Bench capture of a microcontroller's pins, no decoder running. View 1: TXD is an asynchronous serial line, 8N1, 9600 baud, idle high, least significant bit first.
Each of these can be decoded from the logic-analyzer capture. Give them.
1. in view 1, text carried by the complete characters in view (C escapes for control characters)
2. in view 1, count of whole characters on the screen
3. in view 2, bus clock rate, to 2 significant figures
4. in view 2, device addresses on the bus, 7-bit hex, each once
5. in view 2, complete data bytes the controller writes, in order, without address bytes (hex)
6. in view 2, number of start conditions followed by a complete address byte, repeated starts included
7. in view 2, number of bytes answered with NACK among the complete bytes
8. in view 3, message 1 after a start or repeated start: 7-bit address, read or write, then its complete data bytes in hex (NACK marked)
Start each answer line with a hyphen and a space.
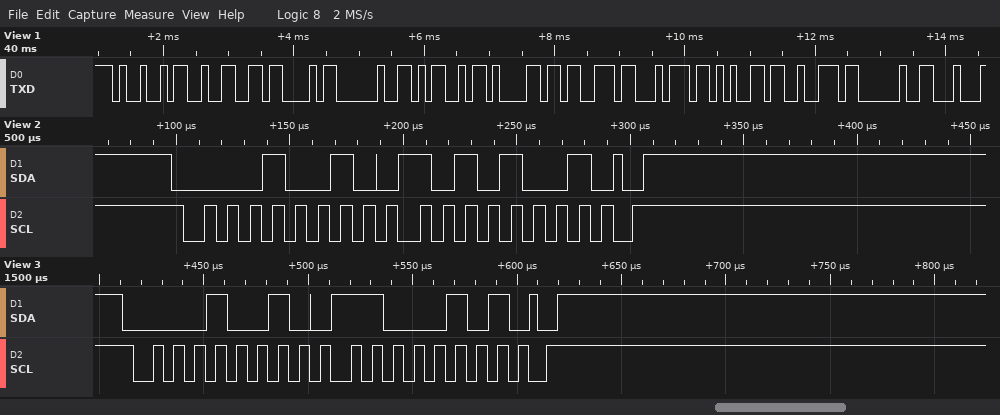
- "I2C Master "
- 11
- 100 kHz
- 0x09
- A9
- 1
- 0
- 0x09 write: C5
